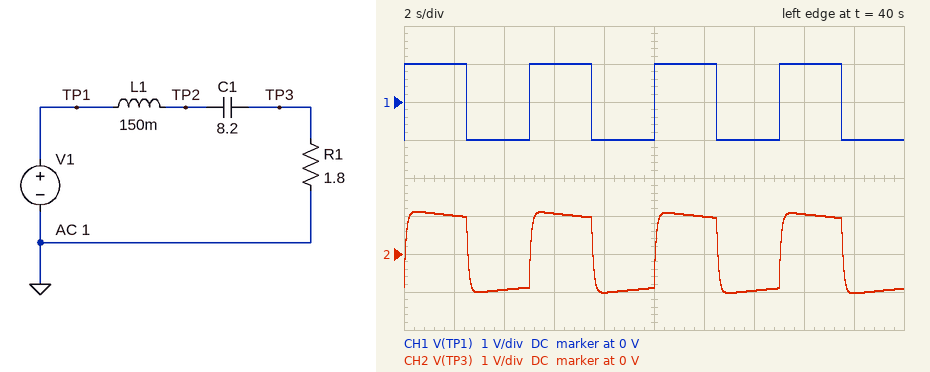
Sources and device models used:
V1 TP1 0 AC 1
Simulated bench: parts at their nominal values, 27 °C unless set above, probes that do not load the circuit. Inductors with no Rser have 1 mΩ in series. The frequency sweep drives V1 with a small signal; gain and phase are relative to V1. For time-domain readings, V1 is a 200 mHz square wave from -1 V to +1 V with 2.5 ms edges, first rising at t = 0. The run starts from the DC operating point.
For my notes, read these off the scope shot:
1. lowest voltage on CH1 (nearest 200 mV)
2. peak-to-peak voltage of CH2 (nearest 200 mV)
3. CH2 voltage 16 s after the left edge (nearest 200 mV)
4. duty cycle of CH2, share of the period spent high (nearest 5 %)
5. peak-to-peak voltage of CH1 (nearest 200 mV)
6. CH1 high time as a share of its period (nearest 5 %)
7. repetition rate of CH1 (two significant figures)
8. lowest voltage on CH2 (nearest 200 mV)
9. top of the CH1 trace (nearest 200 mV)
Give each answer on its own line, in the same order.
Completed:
-1.0 V
2.2 V
1.0 V
50 %
2.0 V
50 %
200 mHz
-1.0 V
1.0 V
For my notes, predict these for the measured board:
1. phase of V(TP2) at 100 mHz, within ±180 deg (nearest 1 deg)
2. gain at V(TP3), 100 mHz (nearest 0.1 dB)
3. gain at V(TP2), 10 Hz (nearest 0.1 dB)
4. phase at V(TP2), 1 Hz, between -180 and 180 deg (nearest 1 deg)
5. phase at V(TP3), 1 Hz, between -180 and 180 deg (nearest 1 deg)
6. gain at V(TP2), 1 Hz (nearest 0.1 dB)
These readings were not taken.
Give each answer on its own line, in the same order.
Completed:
-3 deg
0 dB
-14.5 dB
-28 deg
-27 deg
-1.0 dB
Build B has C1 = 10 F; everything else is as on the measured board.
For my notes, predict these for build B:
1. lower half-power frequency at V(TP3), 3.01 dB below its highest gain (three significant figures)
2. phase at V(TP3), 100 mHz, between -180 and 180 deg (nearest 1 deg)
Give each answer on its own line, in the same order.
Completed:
8.80 mHz
2 deg
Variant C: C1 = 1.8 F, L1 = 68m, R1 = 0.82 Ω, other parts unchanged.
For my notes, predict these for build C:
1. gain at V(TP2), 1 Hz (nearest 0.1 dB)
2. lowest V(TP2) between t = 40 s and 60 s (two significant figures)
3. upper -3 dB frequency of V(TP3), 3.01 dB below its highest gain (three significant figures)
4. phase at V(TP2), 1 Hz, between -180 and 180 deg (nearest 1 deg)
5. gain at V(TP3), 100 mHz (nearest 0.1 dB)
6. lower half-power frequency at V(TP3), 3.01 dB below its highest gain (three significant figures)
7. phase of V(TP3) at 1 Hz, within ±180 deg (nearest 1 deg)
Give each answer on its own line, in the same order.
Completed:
-0.6 dB
-1.1 V
2.02 Hz
-29 deg
-3.1 dB
102 mHz
-22 deg
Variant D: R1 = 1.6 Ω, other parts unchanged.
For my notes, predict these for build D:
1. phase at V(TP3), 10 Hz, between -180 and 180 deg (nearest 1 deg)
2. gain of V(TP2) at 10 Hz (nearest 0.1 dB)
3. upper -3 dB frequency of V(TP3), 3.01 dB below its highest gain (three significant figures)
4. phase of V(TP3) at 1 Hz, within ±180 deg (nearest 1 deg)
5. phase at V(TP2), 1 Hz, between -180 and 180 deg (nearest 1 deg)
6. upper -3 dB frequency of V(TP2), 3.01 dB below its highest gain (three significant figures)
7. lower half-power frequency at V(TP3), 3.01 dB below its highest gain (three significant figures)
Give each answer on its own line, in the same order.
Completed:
-80 deg
-15.5 dB
1.71 Hz
-30 deg
-31 deg
1.69 Hz
12.0 mHz
